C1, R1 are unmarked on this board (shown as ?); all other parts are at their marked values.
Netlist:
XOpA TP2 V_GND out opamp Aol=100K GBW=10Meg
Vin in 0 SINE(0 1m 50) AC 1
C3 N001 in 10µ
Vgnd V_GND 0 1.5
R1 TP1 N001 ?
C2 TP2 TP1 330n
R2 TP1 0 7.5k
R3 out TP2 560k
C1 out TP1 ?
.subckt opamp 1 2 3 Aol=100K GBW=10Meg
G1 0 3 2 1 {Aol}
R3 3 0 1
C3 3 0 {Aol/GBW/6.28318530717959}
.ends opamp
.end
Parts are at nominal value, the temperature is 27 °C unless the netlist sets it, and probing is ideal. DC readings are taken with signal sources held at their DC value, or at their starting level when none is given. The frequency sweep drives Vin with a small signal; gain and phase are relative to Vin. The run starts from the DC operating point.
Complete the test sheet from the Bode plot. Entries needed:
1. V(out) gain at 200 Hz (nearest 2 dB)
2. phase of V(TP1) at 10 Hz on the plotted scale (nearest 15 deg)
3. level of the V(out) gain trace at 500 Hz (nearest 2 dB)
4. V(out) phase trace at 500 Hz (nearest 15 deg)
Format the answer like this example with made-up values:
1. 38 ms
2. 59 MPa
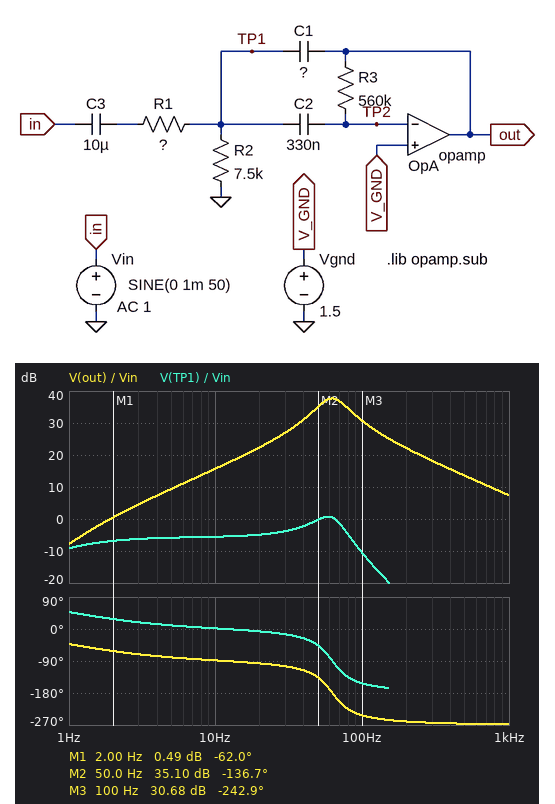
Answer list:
1. 22 dB
2. 0 deg
3. 14 dB
4. -270 deg
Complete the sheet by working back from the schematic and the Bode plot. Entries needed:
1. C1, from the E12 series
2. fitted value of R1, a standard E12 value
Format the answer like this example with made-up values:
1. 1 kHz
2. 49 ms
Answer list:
1. 10 nF
2. 6.8 kΩ
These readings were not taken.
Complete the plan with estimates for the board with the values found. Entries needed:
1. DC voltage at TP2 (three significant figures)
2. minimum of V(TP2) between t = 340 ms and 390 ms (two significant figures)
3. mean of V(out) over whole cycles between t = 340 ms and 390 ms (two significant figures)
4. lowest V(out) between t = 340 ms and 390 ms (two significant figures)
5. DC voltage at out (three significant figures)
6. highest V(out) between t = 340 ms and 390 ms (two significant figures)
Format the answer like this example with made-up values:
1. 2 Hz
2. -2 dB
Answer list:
1. 1.50 V
2. 1.5 V
3. 1.5 V
4. 1.4 V
5. 1.50 V
6. 1.6 V
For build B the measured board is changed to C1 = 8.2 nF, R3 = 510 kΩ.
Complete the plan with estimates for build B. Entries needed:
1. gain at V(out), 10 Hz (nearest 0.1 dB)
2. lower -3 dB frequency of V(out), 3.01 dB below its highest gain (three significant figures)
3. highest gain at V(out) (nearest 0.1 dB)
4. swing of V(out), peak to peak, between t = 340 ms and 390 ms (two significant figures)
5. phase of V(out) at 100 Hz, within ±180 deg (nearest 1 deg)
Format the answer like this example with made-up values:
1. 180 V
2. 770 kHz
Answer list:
1. 14.9 dB
2. 54.7 Hz
3. 37.0 dB
4. 85 mV
5. 131 deg
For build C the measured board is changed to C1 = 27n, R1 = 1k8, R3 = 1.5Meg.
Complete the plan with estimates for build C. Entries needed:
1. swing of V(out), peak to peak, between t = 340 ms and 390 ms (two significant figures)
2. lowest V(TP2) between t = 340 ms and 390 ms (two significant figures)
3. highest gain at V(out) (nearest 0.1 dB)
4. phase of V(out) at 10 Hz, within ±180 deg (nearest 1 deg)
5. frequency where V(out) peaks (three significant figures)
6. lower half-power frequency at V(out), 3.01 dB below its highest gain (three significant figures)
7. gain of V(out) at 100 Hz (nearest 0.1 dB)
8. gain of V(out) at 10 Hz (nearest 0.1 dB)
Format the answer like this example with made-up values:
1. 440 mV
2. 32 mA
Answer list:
1. 250 mV
2. 1.5 V
3. 49.1 dB
4. -86 deg
5. 36.4 Hz
6. 31.1 Hz
7. 31.5 dB
8. 28.4 dB
